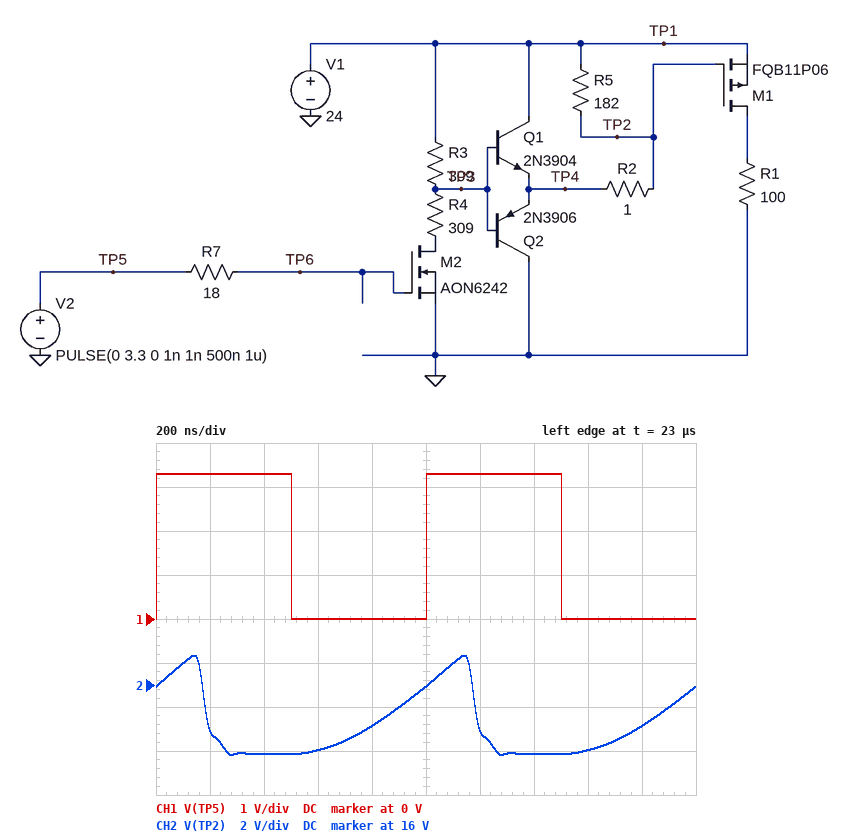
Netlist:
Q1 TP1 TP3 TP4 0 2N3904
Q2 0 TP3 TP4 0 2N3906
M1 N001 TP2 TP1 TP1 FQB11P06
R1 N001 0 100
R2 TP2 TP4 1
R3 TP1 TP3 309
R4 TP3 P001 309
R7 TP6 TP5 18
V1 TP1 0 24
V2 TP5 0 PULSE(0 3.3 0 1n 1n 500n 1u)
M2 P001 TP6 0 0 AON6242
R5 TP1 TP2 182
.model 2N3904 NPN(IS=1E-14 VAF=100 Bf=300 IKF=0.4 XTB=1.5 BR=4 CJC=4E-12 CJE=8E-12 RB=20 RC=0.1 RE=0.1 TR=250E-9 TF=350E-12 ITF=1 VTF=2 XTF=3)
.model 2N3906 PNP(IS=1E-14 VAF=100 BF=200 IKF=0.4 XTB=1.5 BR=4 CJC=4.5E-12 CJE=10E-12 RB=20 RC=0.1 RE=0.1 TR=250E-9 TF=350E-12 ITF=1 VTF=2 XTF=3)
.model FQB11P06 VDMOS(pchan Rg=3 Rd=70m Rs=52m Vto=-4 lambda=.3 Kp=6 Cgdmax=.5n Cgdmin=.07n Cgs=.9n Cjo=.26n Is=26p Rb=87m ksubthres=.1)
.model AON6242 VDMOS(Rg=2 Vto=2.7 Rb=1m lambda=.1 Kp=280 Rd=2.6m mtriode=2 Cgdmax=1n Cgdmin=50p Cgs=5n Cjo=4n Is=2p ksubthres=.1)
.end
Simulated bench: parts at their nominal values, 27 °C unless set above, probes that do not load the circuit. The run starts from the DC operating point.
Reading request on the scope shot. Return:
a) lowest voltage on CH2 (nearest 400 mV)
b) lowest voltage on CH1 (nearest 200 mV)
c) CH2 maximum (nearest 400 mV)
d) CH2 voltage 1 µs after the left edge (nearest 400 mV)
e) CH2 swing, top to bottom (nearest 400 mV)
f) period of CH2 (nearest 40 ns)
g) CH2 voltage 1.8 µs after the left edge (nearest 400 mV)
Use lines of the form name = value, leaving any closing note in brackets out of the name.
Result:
lowest voltage on CH2 = 12.8 V
lowest voltage on CH1 = 0 V
CH2 maximum = 17.2 V
CH2 voltage 1 µs after the left edge = 16.0 V
CH2 swing, top to bottom = 4.4 V
period of CH2 = 1.00 µs
CH2 voltage 1.8 µs after the left edge = 14.0 V
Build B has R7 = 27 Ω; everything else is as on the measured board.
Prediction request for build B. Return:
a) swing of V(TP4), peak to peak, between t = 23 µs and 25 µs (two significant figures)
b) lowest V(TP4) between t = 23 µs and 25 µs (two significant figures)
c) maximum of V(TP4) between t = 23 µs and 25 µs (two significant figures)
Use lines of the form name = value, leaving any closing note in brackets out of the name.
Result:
swing of V(TP4), peak to peak, between t = 23 µs and 25 µs = 5.0 V
lowest V(TP4) between t = 23 µs and 25 µs = 13 V
maximum of V(TP4) between t = 23 µs and 25 µs = 18 V
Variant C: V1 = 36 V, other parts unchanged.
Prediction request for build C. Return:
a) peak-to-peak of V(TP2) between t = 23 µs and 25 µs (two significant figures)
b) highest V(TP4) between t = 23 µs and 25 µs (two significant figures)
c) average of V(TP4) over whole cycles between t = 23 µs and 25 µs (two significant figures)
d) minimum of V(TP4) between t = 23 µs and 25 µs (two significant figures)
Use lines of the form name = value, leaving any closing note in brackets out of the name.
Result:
peak-to-peak of V(TP2) between t = 23 µs and 25 µs = 8.4 V
highest V(TP4) between t = 23 µs and 25 µs = 27 V
average of V(TP4) over whole cycles between t = 23 µs and 25 µs = 21 V
minimum of V(TP4) between t = 23 µs and 25 µs = 19 V
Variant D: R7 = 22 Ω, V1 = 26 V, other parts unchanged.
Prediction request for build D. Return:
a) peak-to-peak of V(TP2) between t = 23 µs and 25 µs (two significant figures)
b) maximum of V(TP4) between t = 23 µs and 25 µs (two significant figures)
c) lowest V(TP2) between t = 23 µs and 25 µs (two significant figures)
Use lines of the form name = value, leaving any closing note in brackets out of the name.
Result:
peak-to-peak of V(TP2) between t = 23 µs and 25 µs = 5.3 V
maximum of V(TP4) between t = 23 µs and 25 µs = 19 V
lowest V(TP2) between t = 23 µs and 25 µs = 14 V
